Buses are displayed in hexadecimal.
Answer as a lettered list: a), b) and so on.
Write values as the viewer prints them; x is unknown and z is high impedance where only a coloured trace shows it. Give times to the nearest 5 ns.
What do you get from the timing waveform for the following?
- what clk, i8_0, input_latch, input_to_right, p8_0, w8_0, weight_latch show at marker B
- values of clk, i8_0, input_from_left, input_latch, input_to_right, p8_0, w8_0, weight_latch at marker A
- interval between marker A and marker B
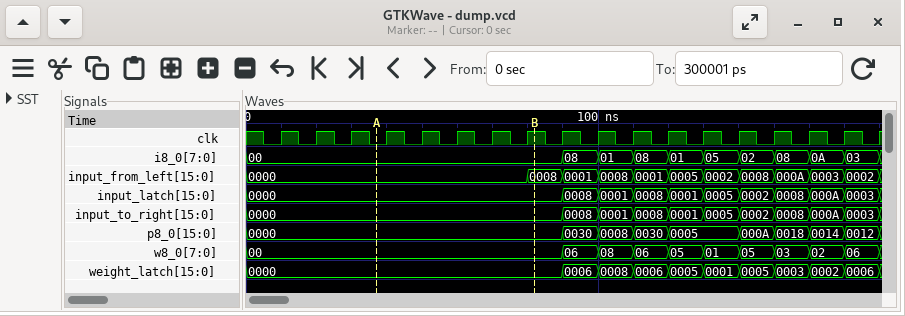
a) clk=1, i8_0=00, input_latch=0000, input_to_right=0000, p8_0=0000, w8_0=00, weight_latch=0000
b) clk=0, i8_0=00, input_from_left=0000, input_latch=0000, input_to_right=0000, p8_0=0000, w8_0=00, weight_latch=0000
c) 45 ns
